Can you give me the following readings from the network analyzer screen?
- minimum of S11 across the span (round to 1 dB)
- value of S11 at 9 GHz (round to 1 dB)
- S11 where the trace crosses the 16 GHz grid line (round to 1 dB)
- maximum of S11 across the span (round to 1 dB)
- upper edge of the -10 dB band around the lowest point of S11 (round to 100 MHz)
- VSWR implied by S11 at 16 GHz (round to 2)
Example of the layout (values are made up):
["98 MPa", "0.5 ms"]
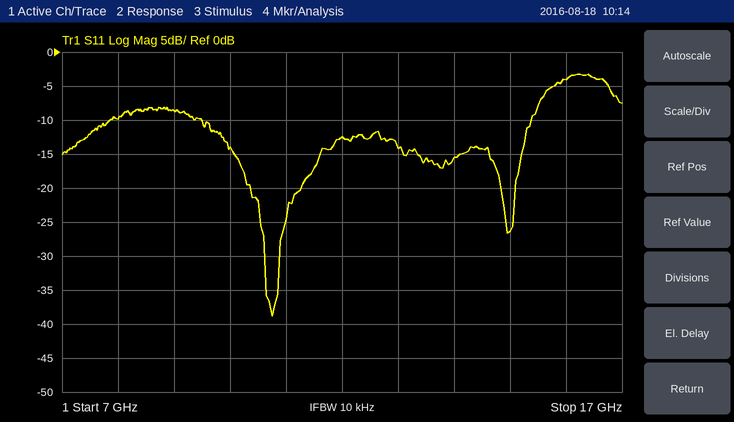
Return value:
["-39 dB", "-9 dB", "-4 dB", "-3 dB", "15.4 GHz", "4"]
